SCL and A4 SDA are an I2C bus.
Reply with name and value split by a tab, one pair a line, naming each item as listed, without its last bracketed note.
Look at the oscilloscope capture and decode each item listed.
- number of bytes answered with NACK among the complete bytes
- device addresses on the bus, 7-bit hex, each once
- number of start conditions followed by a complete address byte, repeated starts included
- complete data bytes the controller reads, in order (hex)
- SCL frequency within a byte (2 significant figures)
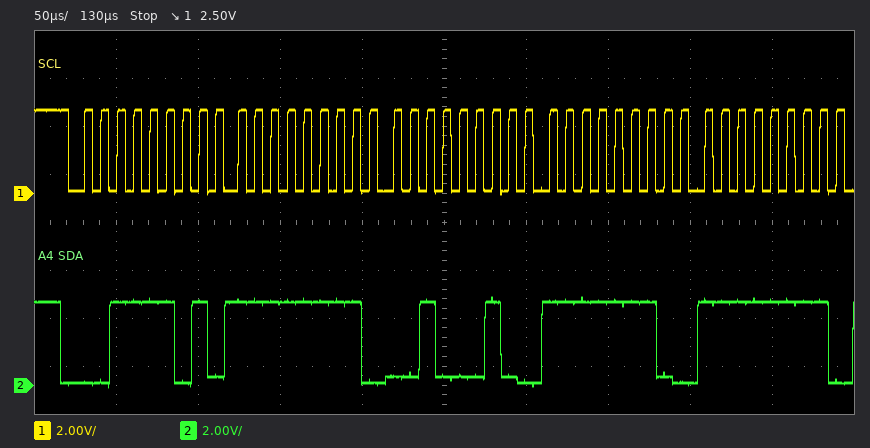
number of bytes answered with NACK among the complete bytes	0
device addresses on the bus, 7-bit hex, each once	0x1E
number of start conditions followed by a complete address byte, repeated starts included	1
complete data bytes the controller reads, in order	FF 22 FE FF
SCL frequency within a byte	100 kHz
